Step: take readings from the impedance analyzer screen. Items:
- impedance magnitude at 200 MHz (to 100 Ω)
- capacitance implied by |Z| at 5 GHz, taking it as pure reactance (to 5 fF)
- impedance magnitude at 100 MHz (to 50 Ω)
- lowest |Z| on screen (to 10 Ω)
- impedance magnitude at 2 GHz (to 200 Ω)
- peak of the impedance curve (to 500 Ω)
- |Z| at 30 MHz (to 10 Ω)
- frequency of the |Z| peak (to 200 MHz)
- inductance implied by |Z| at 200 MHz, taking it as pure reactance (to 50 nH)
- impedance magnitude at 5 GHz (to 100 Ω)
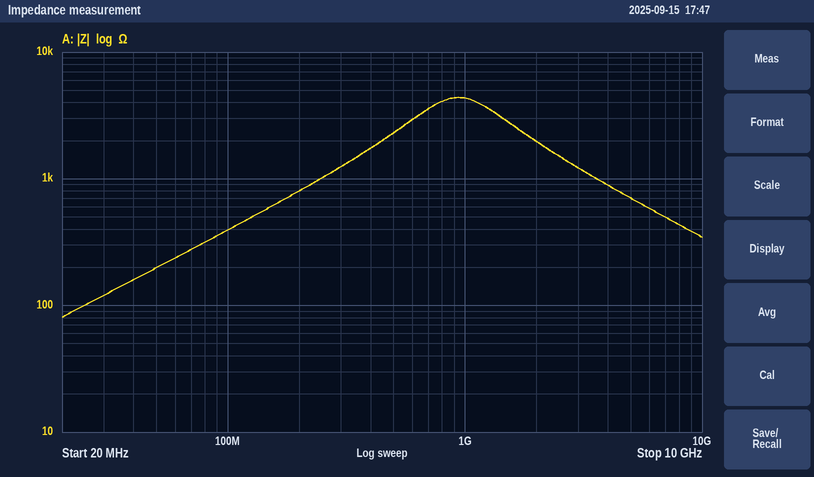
800 Ω
45 fF
400 Ω
80 Ω
2.0 kΩ
4.5 kΩ
120 Ω
1.0 GHz
650 nH
700 Ω
